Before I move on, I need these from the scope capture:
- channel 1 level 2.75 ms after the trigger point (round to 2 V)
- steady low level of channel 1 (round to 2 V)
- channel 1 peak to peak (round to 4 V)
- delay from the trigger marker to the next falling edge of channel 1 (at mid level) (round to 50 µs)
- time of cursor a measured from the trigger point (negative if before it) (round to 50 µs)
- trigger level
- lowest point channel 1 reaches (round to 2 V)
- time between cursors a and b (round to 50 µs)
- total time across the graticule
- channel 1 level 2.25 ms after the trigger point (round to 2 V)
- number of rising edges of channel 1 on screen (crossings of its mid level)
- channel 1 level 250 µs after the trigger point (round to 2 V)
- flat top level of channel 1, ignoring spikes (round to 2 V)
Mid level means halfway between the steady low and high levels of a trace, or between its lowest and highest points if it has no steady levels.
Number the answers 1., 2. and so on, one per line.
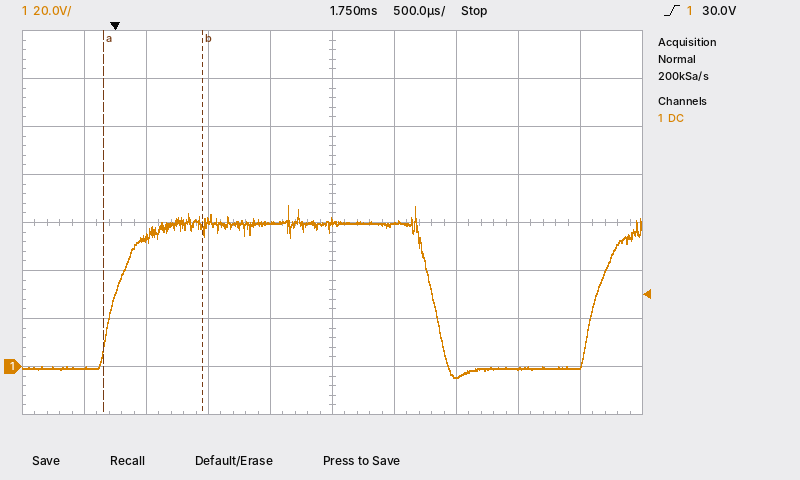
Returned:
1. -4 V
2. 0 V
3. 72 V
4. 2.55 ms
5. -100 µs
6. 30.0 V
7. -4 V
8. 800 µs
9. 5 ms
10. 60 V
11. 2
12. 54 V
13. 60 V
